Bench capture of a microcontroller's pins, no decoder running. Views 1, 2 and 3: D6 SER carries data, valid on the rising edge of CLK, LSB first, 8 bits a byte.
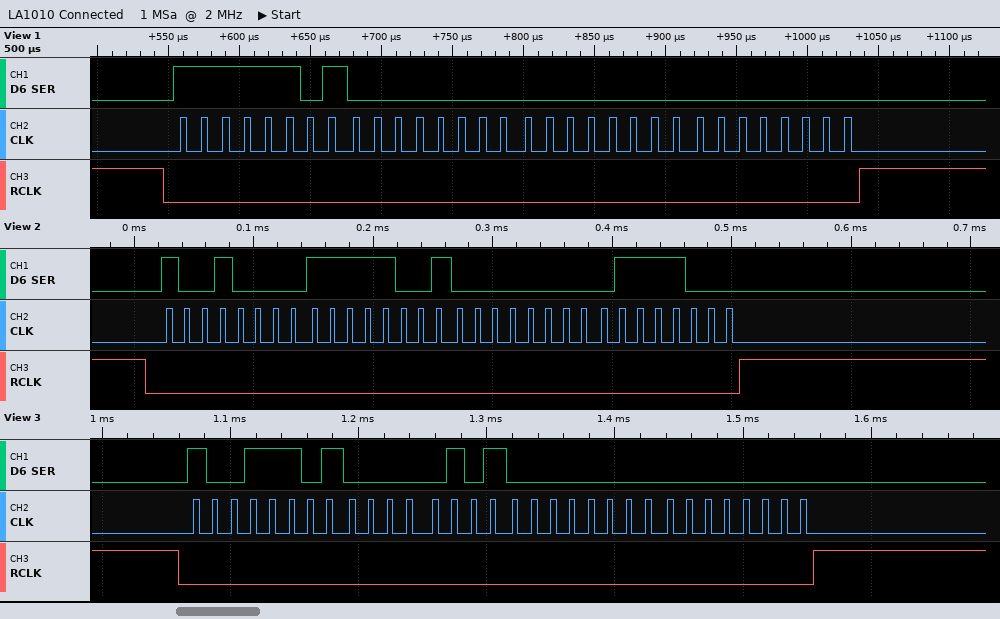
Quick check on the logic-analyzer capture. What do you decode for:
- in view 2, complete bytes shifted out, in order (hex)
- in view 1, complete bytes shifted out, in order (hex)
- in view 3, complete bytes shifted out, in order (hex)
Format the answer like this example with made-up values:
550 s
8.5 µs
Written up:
0x09 0x9F 0x00 0x1E
0xBF 0x00 0x00 0x00
0xB9 0xA0 0x00 0x00
